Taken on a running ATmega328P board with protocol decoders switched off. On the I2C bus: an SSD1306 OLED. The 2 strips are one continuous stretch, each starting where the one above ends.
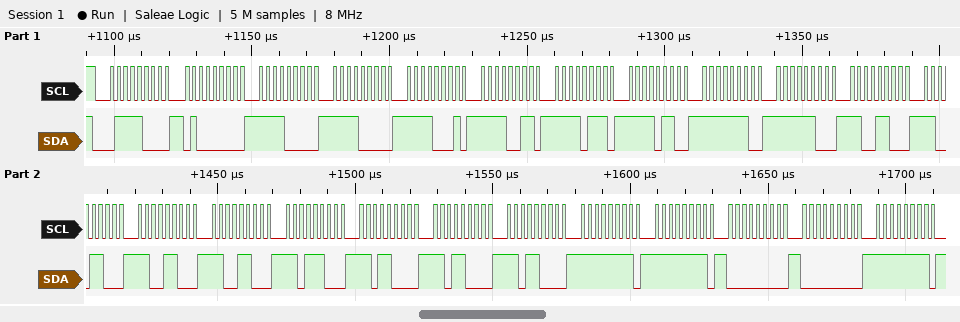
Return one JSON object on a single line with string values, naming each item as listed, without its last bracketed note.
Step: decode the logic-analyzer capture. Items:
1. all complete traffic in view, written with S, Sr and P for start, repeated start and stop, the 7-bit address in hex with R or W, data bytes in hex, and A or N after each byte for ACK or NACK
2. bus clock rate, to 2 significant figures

{"all complete traffic in view, written with S, Sr and P for start, repeated start and stop, the 7-bit address in hex with R or W, data bytes in hex, and A or N after each byte for ACK or NACK": "S 3CW A 40 A F0 A F0 A F1 A F3 A F7 A F6 A FE A FC A CC A CC A CC A CC A DC A D8 A D8 A D8 A FF A FF A 00 A 00 A FF A", "bus clock rate, to 2 significant figures": "400 kHz"}
